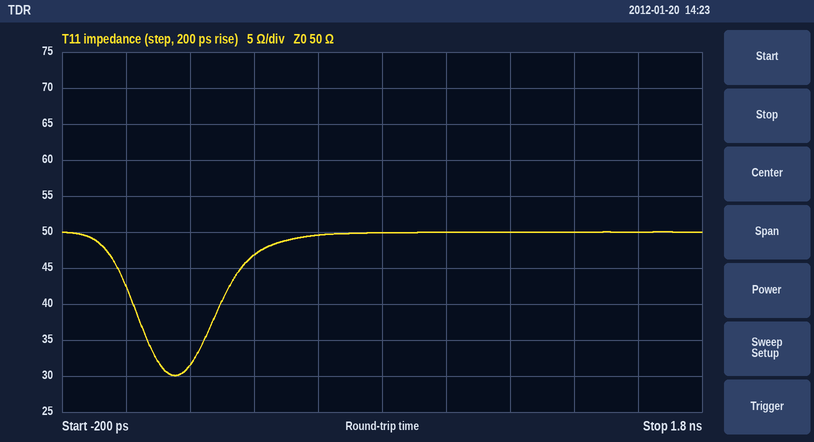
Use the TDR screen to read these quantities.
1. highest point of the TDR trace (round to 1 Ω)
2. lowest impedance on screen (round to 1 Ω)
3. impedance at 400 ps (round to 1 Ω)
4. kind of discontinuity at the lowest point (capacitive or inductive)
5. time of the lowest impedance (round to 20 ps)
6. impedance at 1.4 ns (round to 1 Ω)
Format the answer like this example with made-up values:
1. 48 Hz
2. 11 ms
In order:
1. 50 Ω
2. 30 Ω
3. 47 Ω
4. capacitive
5. 160 ps
6. 50 Ω
